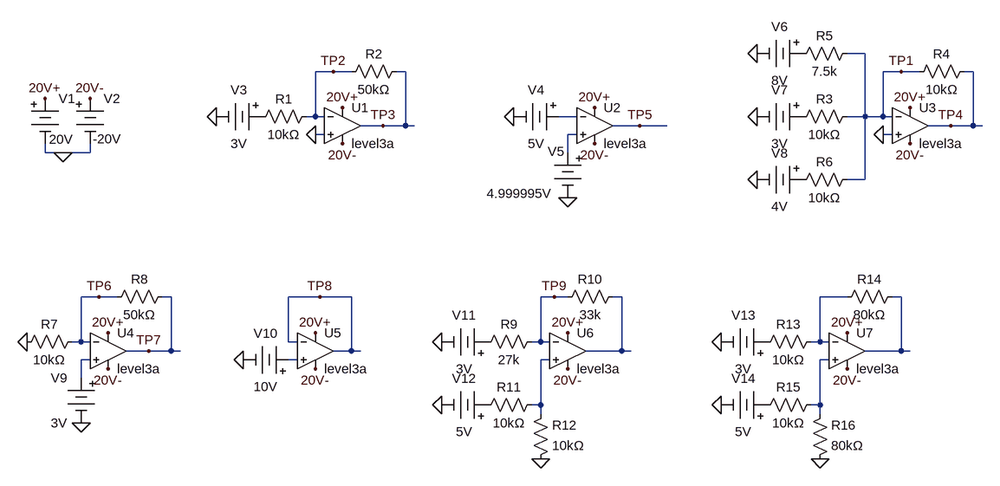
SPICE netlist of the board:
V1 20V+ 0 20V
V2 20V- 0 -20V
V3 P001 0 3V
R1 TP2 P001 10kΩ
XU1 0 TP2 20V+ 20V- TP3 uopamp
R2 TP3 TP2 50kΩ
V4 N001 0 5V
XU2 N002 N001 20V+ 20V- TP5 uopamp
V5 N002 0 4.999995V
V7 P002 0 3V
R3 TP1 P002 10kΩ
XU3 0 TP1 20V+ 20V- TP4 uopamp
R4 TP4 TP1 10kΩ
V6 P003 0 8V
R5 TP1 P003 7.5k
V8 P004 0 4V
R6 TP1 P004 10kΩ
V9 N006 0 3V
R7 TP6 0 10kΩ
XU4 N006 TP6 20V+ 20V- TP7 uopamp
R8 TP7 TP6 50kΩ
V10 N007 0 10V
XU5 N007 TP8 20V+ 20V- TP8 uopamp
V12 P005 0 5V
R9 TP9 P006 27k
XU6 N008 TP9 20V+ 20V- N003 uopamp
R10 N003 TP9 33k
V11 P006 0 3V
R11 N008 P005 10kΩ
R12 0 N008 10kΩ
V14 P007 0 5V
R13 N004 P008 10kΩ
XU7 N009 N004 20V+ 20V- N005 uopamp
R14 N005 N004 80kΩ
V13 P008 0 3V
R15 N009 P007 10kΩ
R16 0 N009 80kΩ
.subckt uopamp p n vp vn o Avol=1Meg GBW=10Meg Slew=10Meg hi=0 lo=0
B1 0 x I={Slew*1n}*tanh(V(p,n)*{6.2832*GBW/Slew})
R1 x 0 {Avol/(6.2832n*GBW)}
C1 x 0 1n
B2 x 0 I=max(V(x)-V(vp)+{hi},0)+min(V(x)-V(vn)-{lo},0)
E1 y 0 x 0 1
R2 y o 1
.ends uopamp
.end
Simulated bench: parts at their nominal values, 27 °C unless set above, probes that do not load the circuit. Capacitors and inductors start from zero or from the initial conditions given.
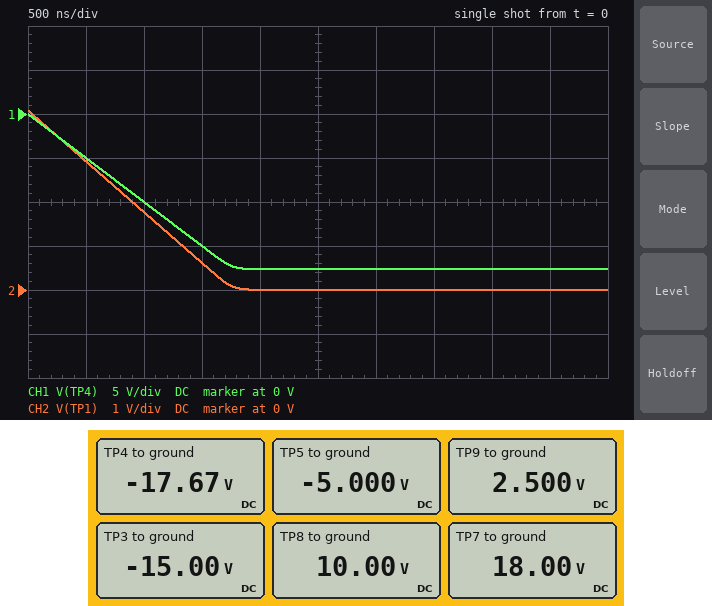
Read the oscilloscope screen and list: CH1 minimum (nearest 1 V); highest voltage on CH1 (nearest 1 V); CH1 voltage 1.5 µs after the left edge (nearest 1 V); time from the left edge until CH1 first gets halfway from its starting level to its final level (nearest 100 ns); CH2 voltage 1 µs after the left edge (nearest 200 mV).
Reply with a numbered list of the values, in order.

1. -18 V
2. 0 V
3. -15 V
4. 900 ns
5. 1.8 V
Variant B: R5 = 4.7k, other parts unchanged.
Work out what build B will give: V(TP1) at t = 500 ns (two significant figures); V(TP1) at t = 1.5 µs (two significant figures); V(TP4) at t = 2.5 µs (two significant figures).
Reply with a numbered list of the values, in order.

1. 3.7 V
2. 1.8 V
3. -20 V
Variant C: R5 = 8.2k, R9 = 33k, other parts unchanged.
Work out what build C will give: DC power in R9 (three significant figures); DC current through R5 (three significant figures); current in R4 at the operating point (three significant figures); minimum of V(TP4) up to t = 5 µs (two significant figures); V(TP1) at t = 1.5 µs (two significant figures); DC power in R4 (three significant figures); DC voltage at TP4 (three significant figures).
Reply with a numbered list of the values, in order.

1. 7.58 µW
2. 976 µA
3. 1.68 mA
4. -17 V
5. 420 mV
6. 28.1 mW
7. -16.8 V
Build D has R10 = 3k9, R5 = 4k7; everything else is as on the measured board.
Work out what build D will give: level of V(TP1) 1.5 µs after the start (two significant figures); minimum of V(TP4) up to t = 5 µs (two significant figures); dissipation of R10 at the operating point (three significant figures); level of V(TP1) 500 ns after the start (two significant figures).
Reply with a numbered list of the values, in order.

1. 1.8 V
2. -20 V
3. 1.34 µW
4. 3.7 V
